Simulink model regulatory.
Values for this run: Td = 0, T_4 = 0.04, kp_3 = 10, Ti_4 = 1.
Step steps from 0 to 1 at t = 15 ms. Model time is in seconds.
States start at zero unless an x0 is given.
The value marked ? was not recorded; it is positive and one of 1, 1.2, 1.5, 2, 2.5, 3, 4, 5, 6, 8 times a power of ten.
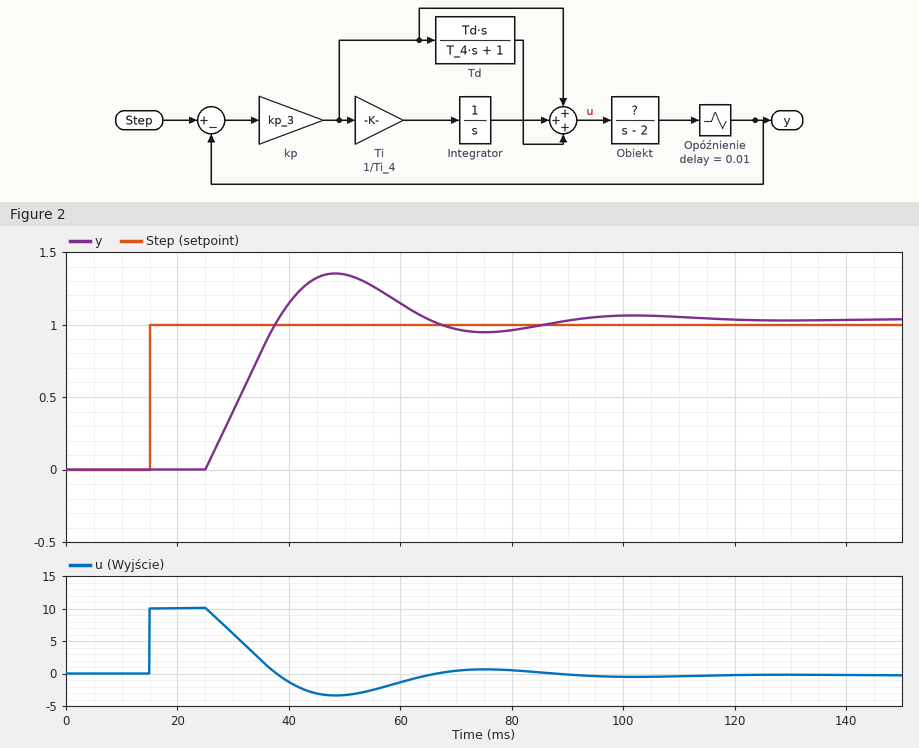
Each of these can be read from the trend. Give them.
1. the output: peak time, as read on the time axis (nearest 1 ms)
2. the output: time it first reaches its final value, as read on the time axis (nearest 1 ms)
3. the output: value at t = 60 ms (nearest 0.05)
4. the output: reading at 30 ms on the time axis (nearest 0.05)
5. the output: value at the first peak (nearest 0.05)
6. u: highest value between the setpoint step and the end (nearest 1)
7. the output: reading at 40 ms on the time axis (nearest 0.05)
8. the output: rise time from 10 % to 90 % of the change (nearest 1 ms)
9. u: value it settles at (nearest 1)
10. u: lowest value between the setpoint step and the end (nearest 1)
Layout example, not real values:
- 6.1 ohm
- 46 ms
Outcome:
- 48 ms
- 38 ms
- 1.15
- 0.40
- 1.35
- 10
- 1.15
- 10 ms
- 0
- -3
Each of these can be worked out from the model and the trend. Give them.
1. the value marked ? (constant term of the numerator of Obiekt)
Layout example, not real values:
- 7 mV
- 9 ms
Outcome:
- 8
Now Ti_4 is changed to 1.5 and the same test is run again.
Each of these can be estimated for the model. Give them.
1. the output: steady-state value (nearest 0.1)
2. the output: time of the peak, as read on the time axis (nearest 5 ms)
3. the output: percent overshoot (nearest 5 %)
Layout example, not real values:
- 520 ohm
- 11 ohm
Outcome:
- 1.0
- 50 ms
- 30 %
